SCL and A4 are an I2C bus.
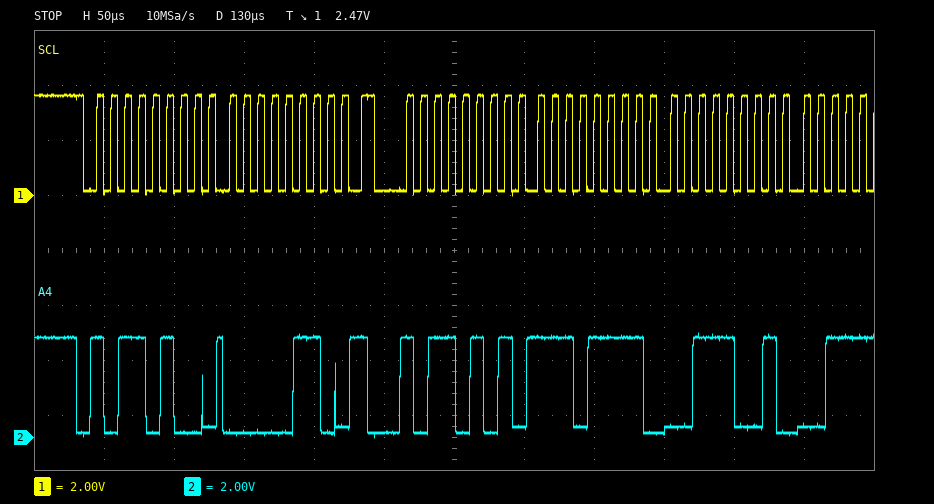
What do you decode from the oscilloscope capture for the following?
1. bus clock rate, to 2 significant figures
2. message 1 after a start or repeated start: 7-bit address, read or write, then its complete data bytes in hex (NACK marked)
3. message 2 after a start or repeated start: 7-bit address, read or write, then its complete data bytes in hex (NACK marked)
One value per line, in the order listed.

100 kHz
0x5A write: 06
0x5A read: EF 39
